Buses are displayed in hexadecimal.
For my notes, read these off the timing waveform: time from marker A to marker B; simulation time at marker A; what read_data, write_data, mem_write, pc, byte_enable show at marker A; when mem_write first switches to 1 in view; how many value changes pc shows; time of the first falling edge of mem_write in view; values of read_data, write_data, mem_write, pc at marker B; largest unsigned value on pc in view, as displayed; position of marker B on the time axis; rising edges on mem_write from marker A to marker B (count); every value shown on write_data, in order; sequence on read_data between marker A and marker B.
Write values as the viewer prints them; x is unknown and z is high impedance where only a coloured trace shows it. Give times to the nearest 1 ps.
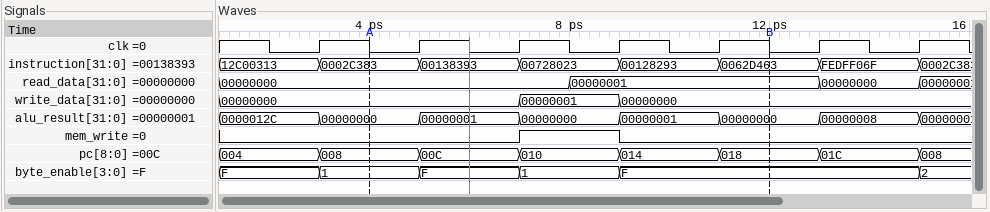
8 ps
4 ps
read_data=00000000, write_data=00000000, mem_write=0, pc=008, byte_enable=1
7 ps
7
9 ps
read_data=00000001, write_data=00000000, mem_write=0, pc=018
01C
12 ps
1
00000000, 00000001, 00000000
00000000, 00000001
